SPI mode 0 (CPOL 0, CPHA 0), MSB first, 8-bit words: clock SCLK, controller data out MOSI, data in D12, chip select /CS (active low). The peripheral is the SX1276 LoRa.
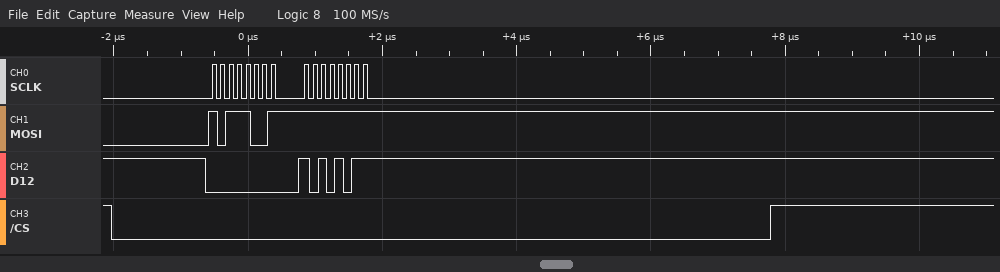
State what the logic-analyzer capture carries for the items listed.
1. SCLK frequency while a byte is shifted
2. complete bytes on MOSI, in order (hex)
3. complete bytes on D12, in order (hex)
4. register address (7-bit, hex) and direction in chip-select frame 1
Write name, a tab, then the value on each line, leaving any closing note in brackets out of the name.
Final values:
SCLK frequency while a byte is shifted	8 MHz
complete bytes on MOSI, in order	B9 FF
complete bytes on D12, in order	00 AB
register address (7-bit, hex) and direction in chip-select frame 1	0x39 write
